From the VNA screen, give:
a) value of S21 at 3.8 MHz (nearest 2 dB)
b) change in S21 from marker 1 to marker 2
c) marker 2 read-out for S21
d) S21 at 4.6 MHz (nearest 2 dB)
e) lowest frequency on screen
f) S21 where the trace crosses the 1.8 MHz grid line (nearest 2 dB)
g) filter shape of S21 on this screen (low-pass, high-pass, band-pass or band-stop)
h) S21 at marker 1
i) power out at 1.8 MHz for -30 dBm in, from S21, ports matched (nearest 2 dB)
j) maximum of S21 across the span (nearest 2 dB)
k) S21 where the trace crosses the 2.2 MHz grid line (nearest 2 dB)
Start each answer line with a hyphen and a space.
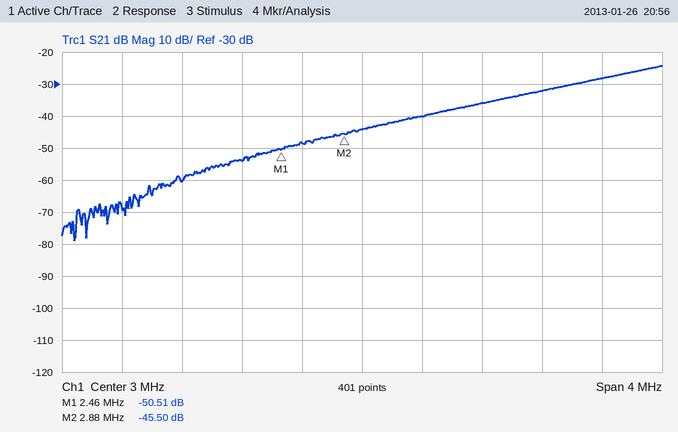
- -36 dB
- 5.01 dB
- -45.50 dB
- -28 dB
- 1 MHz
- -60 dB
- high-pass
- -50.51 dB
- -90 dBm
- -24 dB
- -54 dB
